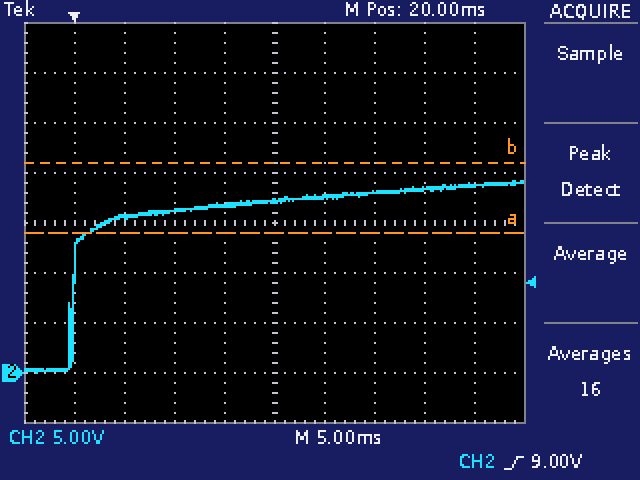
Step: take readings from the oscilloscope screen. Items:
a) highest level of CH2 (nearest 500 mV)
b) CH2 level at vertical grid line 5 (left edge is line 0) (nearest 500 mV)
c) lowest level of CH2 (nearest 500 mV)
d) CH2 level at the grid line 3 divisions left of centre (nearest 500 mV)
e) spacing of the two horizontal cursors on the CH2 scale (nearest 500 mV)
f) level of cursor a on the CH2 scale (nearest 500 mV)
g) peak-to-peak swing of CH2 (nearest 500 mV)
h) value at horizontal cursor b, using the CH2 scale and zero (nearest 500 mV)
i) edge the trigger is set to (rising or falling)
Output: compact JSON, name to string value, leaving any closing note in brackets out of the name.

{"highest level of CH2": "19.0 V", "CH2 level at vertical grid line 5 (left edge is line 0)": "17.0 V", "lowest level of CH2": "0.0 V", "CH2 level at the grid line 3 divisions left of centre": "15.5 V", "spacing of the two horizontal cursors on the CH2 scale": "7.0 V", "level of cursor a on the CH2 scale": "14.0 V", "peak-to-peak swing of CH2": "19.0 V", "value at horizontal cursor b, using the CH2 scale and zero": "21.0 V", "edge the trigger is set to": "rising"}
